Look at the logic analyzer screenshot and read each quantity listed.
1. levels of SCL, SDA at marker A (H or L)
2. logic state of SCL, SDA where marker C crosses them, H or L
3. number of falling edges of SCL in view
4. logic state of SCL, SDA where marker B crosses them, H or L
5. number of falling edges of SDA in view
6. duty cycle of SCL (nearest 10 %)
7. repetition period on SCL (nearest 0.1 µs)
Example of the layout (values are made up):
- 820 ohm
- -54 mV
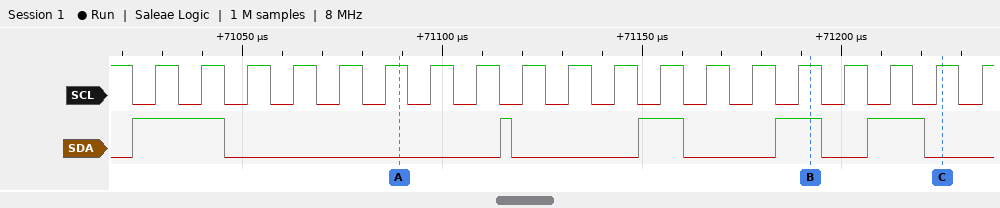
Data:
- SCL=H, SDA=L
- SCL=H, SDA=L
- 19
- SCL=H, SDA=H
- 5
- 50 %
- 11.5 µs
